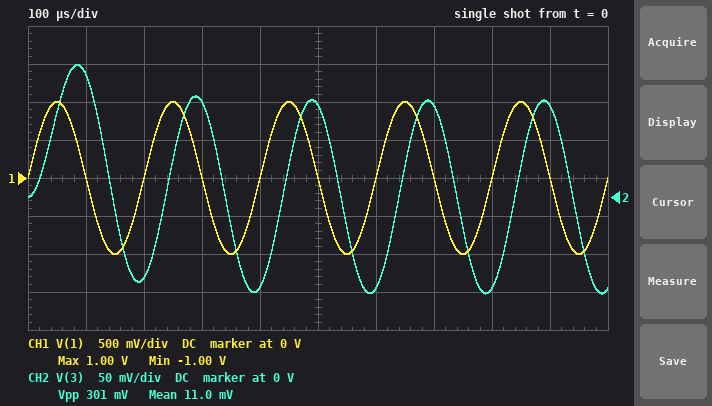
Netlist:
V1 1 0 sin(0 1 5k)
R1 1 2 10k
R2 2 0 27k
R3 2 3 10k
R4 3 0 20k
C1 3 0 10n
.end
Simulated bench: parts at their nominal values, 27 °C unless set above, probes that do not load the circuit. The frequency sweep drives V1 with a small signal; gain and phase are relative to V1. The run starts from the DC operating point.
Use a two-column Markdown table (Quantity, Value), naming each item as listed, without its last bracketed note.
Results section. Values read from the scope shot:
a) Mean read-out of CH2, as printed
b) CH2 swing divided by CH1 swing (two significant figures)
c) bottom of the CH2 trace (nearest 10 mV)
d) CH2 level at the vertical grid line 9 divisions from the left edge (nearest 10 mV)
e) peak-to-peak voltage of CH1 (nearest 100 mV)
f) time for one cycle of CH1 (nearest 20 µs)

| Quantity | Value |
|---|---|
| Mean read-out of CH2, as printed | 11.0 mV |
| CH2 swing divided by CH1 swing | 0.15 |
| bottom of the CH2 trace | -130 mV |
| CH2 level at the vertical grid line 9 divisions from the left edge | 120 mV |
| peak-to-peak voltage of CH1 | 2.0 V |
| time for one cycle of CH1 | 200 µs |
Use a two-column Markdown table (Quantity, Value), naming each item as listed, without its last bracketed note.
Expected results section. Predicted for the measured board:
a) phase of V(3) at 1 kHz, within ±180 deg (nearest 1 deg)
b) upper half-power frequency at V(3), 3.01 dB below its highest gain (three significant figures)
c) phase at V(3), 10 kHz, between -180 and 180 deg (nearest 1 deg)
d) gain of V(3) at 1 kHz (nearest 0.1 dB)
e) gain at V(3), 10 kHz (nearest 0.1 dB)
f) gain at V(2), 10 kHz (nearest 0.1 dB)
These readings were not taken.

| Quantity | Value |
|---|---|
| phase of V(3) at 1 kHz, within ±180 deg | -30 deg |
| upper half-power frequency at V(3), 3.01 dB below its highest gain | 1.72 kHz |
| phase at V(3), 10 kHz, between -180 and 180 deg | -80 deg |
| gain of V(3) at 1 kHz | -9.4 dB |
| gain at V(3), 10 kHz | -23.6 dB |
| gain at V(2), 10 kHz | -7.4 dB |
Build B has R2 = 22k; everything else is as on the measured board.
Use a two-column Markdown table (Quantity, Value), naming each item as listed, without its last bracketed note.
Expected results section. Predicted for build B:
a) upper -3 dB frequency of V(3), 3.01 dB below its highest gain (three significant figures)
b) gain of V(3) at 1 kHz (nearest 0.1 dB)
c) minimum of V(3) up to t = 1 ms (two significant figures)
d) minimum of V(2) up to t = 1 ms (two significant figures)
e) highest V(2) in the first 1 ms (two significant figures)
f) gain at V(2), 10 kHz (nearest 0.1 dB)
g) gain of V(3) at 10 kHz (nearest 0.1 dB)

| Quantity | Value |
|---|---|
| upper -3 dB frequency of V(3), 3.01 dB below its highest gain | 1.74 kHz |
| gain of V(3) at 1 kHz | -9.8 dB |
| minimum of V(3) up to t = 1 ms | -120 mV |
| minimum of V(2) up to t = 1 ms | -430 mV |
| highest V(2) in the first 1 ms | 450 mV |
| gain at V(2), 10 kHz | -7.7 dB |
| gain of V(3) at 10 kHz | -23.9 dB |
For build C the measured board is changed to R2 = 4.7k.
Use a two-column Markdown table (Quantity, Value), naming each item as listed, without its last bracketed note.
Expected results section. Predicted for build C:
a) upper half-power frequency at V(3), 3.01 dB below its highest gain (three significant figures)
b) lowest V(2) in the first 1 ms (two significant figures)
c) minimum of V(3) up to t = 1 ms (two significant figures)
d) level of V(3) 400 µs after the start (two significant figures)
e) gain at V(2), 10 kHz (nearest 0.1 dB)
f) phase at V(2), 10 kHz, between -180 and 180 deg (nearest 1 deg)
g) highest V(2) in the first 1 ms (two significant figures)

| Quantity | Value |
|---|---|
| upper half-power frequency at V(3), 3.01 dB below its highest gain | 2.00 kHz |
| lowest V(2) in the first 1 ms | -250 mV |
| minimum of V(3) up to t = 1 ms | -72 mV |
| level of V(3) 400 µs after the start | -66 mV |
| gain at V(2), 10 kHz | -12.2 dB |
| phase at V(2), 10 kHz, between -180 and 180 deg | -2 deg |
| highest V(2) in the first 1 ms | 260 mV |
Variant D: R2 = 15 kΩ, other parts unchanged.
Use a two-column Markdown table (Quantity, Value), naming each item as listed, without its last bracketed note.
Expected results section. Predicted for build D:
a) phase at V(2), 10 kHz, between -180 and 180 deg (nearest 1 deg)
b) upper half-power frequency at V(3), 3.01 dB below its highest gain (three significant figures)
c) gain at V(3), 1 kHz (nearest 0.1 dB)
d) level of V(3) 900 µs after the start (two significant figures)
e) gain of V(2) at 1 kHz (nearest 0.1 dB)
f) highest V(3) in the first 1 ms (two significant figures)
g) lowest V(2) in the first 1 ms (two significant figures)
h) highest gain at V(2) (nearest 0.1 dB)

| Quantity | Value |
|---|---|
| phase at V(2), 10 kHz, between -180 and 180 deg | -3 deg |
| upper half-power frequency at V(3), 3.01 dB below its highest gain | 1.79 kHz |
| gain at V(3), 1 kHz | -10.7 dB |
| level of V(3) 900 µs after the start | 110 mV |
| gain of V(2) at 1 kHz | -6.5 dB |
| highest V(3) in the first 1 ms | 150 mV |
| lowest V(2) in the first 1 ms | -390 mV |
| highest gain at V(2) | -6.0 dB |
